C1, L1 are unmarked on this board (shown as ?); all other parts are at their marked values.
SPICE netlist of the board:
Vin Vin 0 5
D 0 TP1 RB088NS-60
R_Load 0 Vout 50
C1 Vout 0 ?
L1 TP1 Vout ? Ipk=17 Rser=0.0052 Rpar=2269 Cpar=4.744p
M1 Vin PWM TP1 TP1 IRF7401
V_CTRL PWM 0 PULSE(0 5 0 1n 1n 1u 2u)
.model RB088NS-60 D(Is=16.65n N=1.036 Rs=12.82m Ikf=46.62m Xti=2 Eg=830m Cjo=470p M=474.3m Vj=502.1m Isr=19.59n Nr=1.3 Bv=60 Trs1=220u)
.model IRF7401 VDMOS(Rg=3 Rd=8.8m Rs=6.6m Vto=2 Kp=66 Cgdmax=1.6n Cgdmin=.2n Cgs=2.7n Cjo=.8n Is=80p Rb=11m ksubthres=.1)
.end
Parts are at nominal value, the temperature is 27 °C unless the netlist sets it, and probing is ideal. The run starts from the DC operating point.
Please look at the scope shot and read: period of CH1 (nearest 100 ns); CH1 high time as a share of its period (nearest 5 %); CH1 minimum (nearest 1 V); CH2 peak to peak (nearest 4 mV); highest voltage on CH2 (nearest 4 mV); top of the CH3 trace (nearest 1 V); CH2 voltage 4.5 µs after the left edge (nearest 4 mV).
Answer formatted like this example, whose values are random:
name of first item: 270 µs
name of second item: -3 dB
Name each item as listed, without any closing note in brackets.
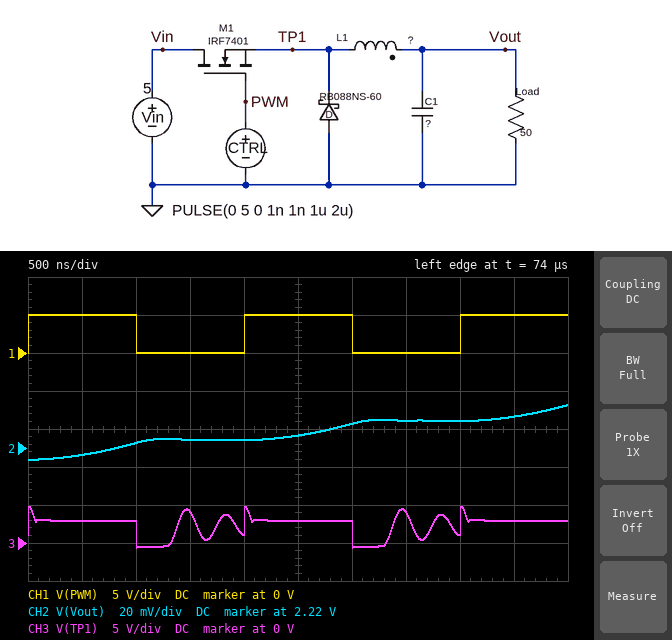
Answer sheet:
period of CH1: 2.0 µs
CH1 high time as a share of its period: 50 %
CH1 minimum: 0 V
CH2 peak to peak: 28 mV
highest voltage on CH2: 2.244 V
top of the CH3 trace: 5 V
CH2 voltage 4.5 µs after the left edge: 2.236 V
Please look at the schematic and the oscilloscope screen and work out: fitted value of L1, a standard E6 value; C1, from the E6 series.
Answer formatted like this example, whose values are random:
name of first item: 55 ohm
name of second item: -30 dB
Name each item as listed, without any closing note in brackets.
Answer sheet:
fitted value of L1, a standard E6 value: 1 µH
C1, from the E6 series: 47 µF
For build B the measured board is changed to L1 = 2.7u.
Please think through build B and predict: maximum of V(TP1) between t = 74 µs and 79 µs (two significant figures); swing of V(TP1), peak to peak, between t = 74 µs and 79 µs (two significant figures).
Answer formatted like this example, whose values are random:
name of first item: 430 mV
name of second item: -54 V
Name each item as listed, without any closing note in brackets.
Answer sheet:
maximum of V(TP1) between t = 74 µs and 79 µs: 4.2 V
swing of V(TP1), peak to peak, between t = 74 µs and 79 µs: 4.8 V
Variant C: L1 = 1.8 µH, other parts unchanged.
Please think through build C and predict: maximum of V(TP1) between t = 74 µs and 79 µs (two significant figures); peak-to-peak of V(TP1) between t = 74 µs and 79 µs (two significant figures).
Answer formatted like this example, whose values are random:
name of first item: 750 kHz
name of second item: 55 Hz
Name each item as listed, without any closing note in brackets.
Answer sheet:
maximum of V(TP1) between t = 74 µs and 79 µs: 5.6 V
peak-to-peak of V(TP1) between t = 74 µs and 79 µs: 6.1 V
